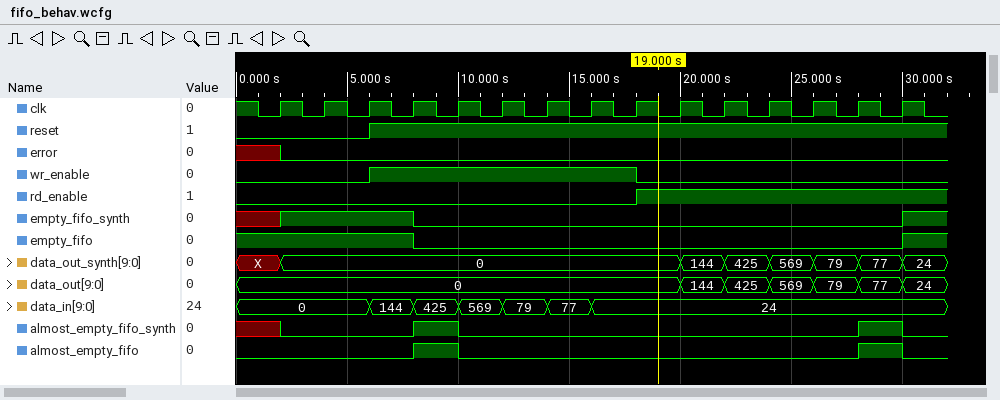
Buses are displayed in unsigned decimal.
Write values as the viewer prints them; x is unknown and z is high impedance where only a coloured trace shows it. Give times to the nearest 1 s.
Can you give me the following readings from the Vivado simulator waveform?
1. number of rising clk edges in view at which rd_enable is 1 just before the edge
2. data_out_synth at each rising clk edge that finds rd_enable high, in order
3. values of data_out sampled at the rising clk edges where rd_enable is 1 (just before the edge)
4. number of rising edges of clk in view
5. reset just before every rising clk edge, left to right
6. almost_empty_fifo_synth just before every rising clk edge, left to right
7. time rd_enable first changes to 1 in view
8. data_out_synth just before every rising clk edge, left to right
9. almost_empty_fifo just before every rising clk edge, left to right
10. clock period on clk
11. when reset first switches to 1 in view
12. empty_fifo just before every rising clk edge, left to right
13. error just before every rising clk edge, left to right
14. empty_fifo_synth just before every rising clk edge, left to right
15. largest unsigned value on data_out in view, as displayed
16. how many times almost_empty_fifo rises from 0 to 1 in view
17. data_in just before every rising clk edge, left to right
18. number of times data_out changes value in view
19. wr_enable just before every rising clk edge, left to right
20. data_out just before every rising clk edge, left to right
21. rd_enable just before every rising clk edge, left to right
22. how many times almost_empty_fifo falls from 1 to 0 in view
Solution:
6
0, 144, 425, 569, 79, 77
0, 144, 425, 569, 79, 77
15
0 0 0 1 1 1 1 1 1 1 1 1 1 1 1
x 0 0 0 1 0 0 0 0 0 0 0 0 0 1
18 s
X, 0, 0, 0, 0, 0, 0, 0, 0, 0, 144, 425, 569, 79, 77
0 0 0 0 1 0 0 0 0 0 0 0 0 0 1
2 s
6 s
1 1 1 1 0 0 0 0 0 0 0 0 0 0 0
x 0 0 0 0 0 0 0 0 0 0 0 0 0 0
x 1 1 1 0 0 0 0 0 0 0 0 0 0 0
569
2
0, 0, 0, 144, 425, 569, 79, 77, 24, 24, 24, 24, 24, 24, 24
6
0 0 0 1 1 1 1 1 1 0 0 0 0 0 0
0, 0, 0, 0, 0, 0, 0, 0, 0, 0, 144, 425, 569, 79, 77
0 0 0 0 0 0 0 0 0 1 1 1 1 1 1
2
